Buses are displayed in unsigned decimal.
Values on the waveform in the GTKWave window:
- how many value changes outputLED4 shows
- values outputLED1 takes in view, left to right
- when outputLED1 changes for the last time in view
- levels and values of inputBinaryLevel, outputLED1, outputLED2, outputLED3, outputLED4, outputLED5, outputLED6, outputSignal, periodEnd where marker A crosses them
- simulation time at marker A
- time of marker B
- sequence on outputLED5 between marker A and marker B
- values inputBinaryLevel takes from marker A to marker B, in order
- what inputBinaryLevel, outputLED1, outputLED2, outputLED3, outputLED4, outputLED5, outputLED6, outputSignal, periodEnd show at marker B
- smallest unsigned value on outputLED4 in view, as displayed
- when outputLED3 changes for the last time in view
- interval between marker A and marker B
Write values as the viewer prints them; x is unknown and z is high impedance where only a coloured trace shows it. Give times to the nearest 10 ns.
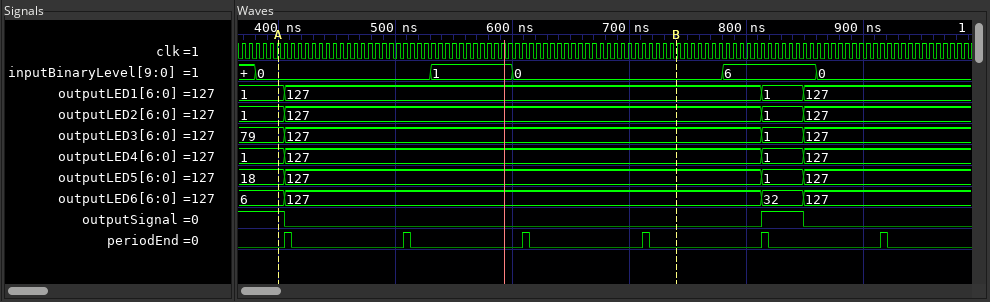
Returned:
3
1, 127, 1, 127
850 ns
inputBinaryLevel=0, outputLED1=1, outputLED2=1, outputLED3=79, outputLED4=1, outputLED5=18, outputLED6=6, outputSignal=1, periodEnd=0
400 ns
740 ns
18, 127
0, 1, 0
inputBinaryLevel=0, outputLED1=127, outputLED2=127, outputLED3=127, outputLED4=127, outputLED5=127, outputLED6=127, outputSignal=0, periodEnd=0
1
850 ns
340 ns
